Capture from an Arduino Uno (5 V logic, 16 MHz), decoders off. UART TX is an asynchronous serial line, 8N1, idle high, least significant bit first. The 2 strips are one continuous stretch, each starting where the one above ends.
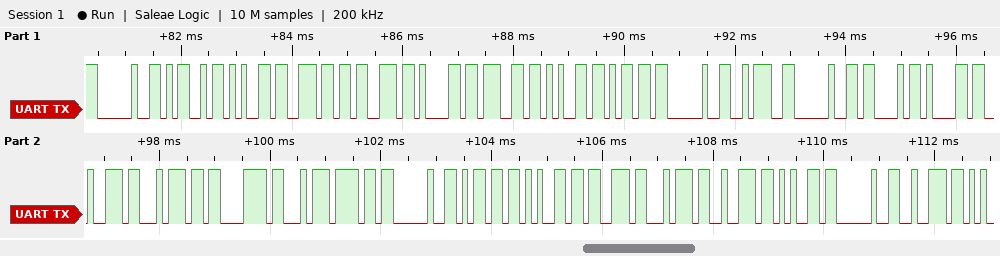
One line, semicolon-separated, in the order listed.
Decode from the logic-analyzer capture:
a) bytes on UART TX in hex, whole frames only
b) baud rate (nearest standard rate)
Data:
20 4D 65 6E 73 61 67 65 6D 20 3A 20 43 61 72 74 C3 A3 6F 20 6D 65 73 74 72 65 20 72; 9600 baud
